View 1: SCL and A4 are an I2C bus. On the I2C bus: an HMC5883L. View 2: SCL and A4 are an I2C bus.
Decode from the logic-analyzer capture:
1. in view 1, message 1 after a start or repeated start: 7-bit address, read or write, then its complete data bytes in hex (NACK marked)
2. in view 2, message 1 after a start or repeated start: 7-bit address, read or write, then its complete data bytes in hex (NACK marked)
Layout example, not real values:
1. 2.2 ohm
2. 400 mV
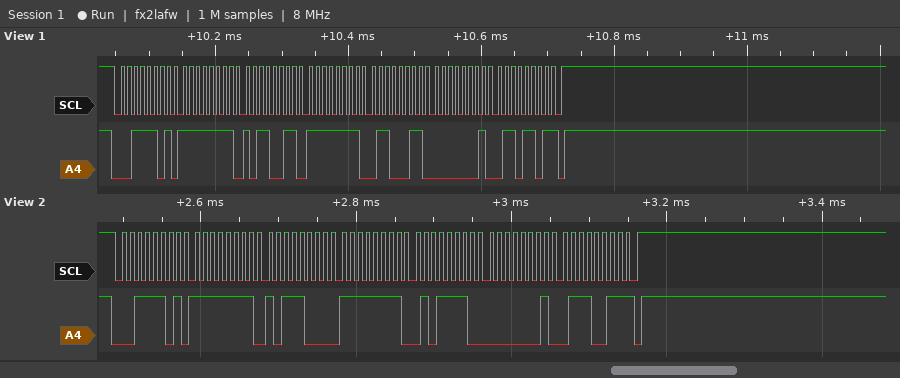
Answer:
1. 0x1E read: FF B3 FF 63 01 6D NACK
2. 0x1E read: FF B8 FF 5E 01 73 NACK
